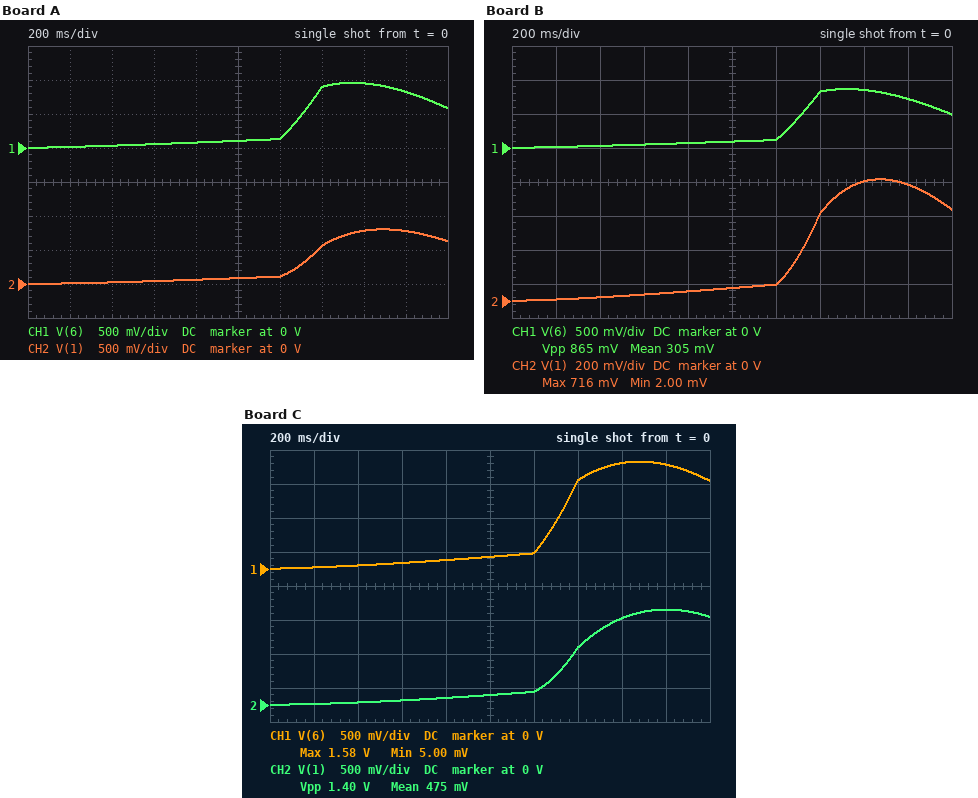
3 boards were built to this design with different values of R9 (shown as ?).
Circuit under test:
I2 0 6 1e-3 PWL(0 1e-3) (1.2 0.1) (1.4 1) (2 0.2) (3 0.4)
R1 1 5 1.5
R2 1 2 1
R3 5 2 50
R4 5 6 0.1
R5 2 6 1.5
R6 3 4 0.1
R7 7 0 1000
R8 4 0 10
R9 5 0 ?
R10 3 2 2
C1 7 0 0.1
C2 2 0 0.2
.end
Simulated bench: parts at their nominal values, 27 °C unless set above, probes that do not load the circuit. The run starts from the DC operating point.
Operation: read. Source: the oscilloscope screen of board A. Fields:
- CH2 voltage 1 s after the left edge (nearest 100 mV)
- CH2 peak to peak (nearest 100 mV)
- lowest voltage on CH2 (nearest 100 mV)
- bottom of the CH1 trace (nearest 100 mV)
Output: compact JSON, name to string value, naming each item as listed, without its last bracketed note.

{"CH2 voltage 1 s after the left edge": "100 mV", "CH2 peak to peak": "800 mV", "lowest voltage on CH2": "0 V", "bottom of the CH1 trace": "0 V"}
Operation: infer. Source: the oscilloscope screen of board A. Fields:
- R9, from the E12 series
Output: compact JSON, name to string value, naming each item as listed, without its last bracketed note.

{"R9, from the E12 series": "1.8 Ω"}
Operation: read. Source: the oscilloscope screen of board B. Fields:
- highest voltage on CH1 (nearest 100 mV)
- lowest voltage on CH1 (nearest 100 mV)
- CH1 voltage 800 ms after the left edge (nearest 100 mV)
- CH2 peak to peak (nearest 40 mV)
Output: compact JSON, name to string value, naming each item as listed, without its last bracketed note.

{"highest voltage on CH1": "900 mV", "lowest voltage on CH1": "0 V", "CH1 voltage 800 ms after the left edge": "100 mV", "CH2 peak to peak": "720 mV"}
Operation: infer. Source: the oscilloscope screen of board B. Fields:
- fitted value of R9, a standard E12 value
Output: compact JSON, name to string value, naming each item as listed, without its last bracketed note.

{"fitted value of R9, a standard E12 value": "1.5 Ω"}
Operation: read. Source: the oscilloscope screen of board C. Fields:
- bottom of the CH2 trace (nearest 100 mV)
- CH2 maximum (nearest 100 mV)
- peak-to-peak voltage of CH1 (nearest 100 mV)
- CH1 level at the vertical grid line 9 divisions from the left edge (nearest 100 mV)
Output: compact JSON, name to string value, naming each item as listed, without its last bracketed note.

{"bottom of the CH2 trace": "0 V", "CH2 maximum": "1.4 V", "peak-to-peak voltage of CH1": "1.6 V", "CH1 level at the vertical grid line 9 divisions from the left edge": "1.5 V"}
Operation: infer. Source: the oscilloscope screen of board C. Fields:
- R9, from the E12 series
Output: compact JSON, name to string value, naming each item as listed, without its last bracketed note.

{"R9, from the E12 series": "5.6 Ω"}
